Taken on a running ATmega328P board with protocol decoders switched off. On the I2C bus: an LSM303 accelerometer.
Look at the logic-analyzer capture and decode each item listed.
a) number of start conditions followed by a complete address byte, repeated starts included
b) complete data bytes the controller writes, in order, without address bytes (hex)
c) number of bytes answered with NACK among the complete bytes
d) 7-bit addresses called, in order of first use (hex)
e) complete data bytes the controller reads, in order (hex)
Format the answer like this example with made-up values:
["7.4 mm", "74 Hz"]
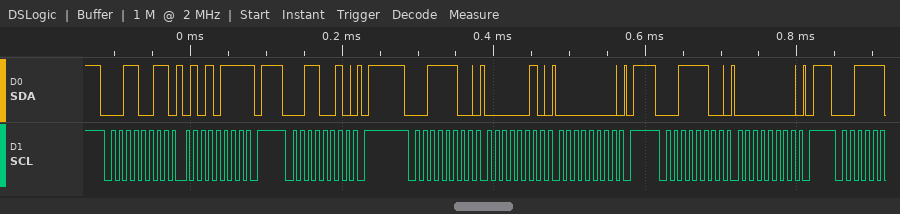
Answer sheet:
["4", "02 00 00", "1", "0x19 0x1E", "57"]
